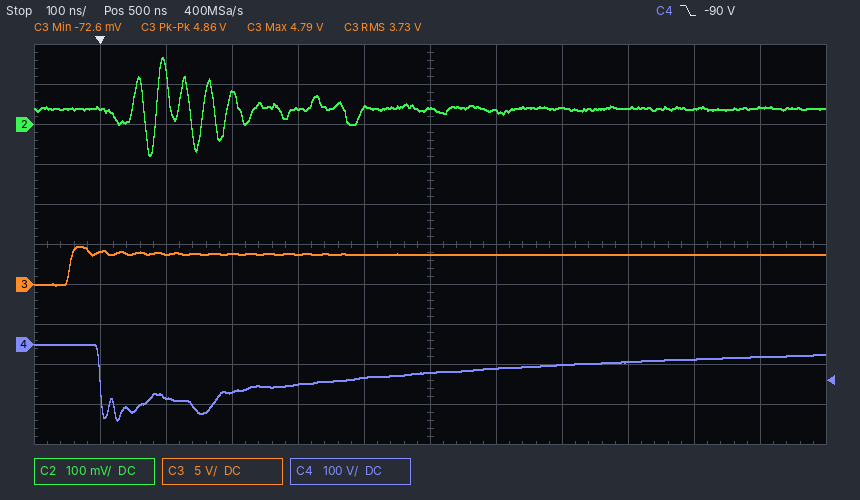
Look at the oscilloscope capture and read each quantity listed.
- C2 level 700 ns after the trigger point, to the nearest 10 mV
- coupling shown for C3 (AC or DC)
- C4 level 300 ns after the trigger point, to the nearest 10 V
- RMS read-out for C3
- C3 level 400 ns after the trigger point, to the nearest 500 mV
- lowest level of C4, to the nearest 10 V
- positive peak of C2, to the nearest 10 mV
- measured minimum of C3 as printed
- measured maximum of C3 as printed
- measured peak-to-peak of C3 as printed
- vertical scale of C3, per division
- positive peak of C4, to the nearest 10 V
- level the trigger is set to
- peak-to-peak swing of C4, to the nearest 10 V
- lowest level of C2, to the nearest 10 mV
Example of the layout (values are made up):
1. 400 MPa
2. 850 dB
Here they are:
1. 40 mV
2. DC
3. -100 V
4. 3.73 V
5. 4.0 V
6. -190 V
7. 170 mV
8. -72.6 mV
9. 4.79 V
10. 4.86 V
11. 5 V
12. 0 V
13. -90 V
14. 190 V
15. -80 mV
